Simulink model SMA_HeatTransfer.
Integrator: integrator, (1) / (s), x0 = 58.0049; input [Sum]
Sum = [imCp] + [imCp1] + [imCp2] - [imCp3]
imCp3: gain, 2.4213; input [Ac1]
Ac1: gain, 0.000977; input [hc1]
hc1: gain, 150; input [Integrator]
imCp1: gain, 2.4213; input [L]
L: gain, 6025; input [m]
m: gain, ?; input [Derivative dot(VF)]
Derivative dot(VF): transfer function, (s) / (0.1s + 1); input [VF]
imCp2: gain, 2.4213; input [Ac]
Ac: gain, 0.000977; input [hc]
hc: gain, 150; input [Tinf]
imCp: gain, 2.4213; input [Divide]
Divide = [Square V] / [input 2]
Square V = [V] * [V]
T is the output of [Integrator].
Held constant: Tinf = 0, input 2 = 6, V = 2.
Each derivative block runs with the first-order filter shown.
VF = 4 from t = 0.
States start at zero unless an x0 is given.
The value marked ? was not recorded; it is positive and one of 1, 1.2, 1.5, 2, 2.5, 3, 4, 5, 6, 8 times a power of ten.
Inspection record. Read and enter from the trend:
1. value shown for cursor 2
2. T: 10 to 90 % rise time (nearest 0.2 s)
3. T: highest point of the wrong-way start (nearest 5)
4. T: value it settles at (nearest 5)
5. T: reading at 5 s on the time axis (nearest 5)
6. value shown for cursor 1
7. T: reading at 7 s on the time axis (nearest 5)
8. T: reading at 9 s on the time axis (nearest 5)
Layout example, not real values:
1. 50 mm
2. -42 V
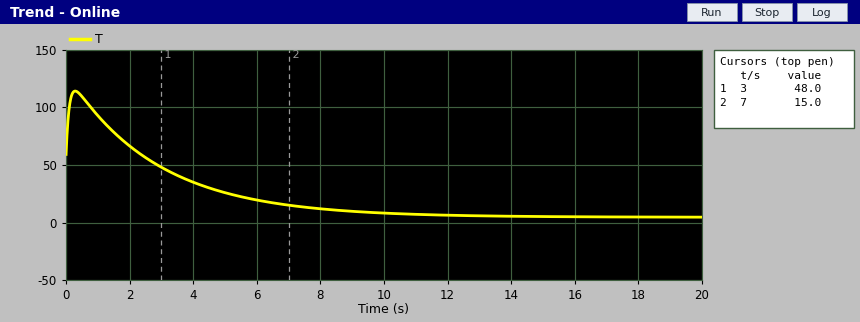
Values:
1. 15.0
2. 6.2 s
3. 115
4. 5
5. 25
6. 48.0
7. 15
8. 10
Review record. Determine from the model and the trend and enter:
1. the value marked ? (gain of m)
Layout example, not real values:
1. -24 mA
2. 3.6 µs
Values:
1. 0.0012
